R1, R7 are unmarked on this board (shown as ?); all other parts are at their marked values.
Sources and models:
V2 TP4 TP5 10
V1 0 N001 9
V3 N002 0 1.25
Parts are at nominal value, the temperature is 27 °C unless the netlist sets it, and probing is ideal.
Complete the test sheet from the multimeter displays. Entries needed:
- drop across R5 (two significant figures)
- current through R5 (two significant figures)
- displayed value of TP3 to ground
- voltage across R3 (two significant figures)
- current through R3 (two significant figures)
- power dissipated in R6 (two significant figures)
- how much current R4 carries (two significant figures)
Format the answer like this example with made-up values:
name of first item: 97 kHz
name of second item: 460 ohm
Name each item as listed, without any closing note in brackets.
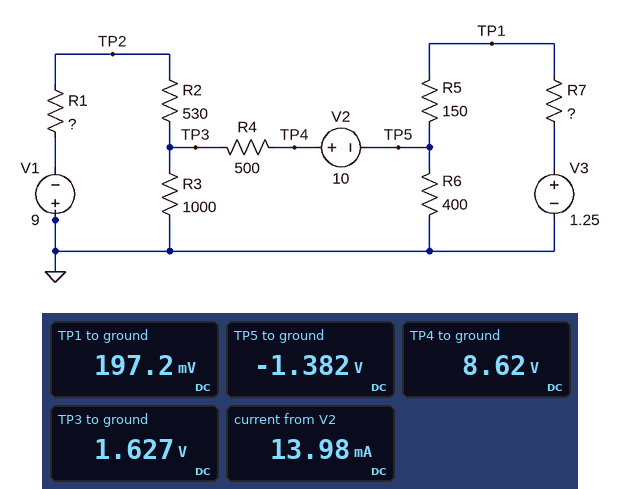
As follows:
drop across R5: 1.6 V
current through R5: 11 mA
displayed value of TP3 to ground: 1.627 V
voltage across R3: 1.6 V
current through R3: 1.6 mA
power dissipated in R6: 4.8 mW
how much current R4 carries: 14 mA
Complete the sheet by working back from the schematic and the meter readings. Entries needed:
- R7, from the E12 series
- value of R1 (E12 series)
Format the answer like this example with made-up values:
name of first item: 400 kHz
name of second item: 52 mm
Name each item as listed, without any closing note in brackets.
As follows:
R7, from the E12 series: 100 Ω
value of R1: 330 Ω
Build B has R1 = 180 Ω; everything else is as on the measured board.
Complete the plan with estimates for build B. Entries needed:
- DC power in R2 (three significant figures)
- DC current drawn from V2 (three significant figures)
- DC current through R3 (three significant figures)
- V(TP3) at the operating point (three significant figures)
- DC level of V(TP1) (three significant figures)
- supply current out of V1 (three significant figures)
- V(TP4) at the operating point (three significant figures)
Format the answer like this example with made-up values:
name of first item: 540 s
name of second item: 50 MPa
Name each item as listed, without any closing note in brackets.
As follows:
DC power in R2: 104 mW
DC current drawn from V2: 15.0 mA
DC current through R3: 964 µA
V(TP3) at the operating point: 964 mV
DC level of V(TP1): 135 mV
supply current out of V1: 14.0 mA
V(TP4) at the operating point: 8.46 V
